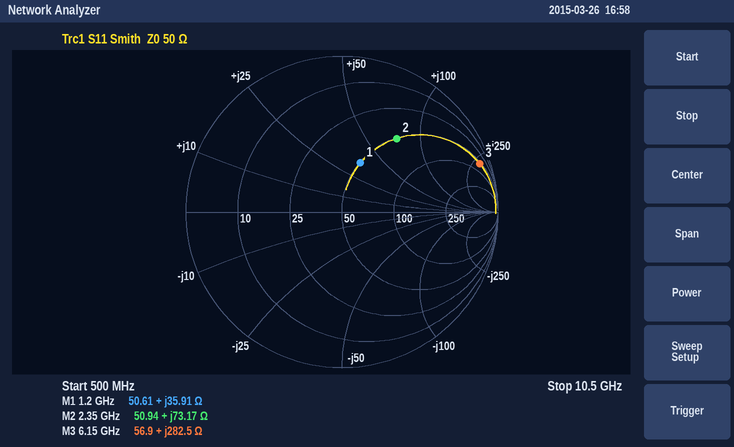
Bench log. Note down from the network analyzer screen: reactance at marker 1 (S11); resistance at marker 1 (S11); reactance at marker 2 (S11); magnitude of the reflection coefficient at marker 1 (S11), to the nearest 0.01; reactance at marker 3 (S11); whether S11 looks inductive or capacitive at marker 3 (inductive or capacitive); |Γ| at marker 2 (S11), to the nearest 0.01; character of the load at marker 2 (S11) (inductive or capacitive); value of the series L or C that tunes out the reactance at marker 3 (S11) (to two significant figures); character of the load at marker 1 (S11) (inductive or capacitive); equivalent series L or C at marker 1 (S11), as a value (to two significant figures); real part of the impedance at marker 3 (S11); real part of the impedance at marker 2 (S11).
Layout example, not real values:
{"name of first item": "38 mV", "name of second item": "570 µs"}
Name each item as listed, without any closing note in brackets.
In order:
{"reactance at marker 1": "+35.91 Ω", "resistance at marker 1": "50.61 Ω", "reactance at marker 2": "+73.17 Ω", "magnitude of the reflection coefficient at marker 1 (S11), to the nearest 0.01": "0.34", "reactance at marker 3": "+282.5 Ω", "whether S11 looks inductive or capacitive at marker 3": "inductive", "|Γ| at marker 2 (S11), to the nearest 0.01": "0.59", "character of the load at marker 2 (S11)": "inductive", "value of the series L or C that tunes out the reactance at marker 3 (S11)": "92 fF", "character of the load at marker 1 (S11)": "inductive", "equivalent series L or C at marker 1 (S11), as a value": "4.8 nH", "real part of the impedance at marker 3": "56.9 Ω", "real part of the impedance at marker 2": "50.94 Ω"}
